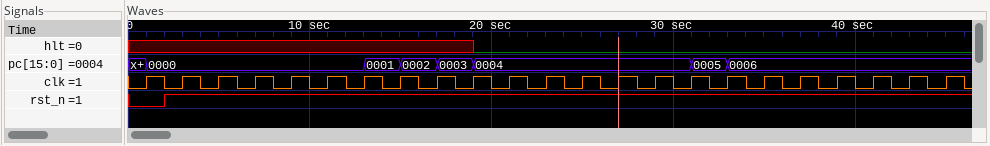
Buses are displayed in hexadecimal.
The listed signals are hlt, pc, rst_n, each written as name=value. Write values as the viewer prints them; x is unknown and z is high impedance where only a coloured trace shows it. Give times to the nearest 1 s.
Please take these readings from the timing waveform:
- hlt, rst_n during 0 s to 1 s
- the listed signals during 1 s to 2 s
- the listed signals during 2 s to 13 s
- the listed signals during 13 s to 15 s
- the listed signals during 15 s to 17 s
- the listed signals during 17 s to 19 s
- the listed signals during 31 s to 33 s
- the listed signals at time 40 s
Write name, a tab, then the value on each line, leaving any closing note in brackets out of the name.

hlt, rst_n during 0 s to 1 s	hlt=x, rst_n=0
the listed signals during 1 s to 2 s	hlt=x, pc=0000, rst_n=0
the listed signals during 2 s to 13 s	hlt=x, pc=0000, rst_n=1
the listed signals during 13 s to 15 s	hlt=x, pc=0001, rst_n=1
the listed signals during 15 s to 17 s	hlt=x, pc=0002, rst_n=1
the listed signals during 17 s to 19 s	hlt=x, pc=0003, rst_n=1
the listed signals during 31 s to 33 s	hlt=0, pc=0005, rst_n=1
the listed signals at time 40 s	hlt=0, pc=0006, rst_n=1
